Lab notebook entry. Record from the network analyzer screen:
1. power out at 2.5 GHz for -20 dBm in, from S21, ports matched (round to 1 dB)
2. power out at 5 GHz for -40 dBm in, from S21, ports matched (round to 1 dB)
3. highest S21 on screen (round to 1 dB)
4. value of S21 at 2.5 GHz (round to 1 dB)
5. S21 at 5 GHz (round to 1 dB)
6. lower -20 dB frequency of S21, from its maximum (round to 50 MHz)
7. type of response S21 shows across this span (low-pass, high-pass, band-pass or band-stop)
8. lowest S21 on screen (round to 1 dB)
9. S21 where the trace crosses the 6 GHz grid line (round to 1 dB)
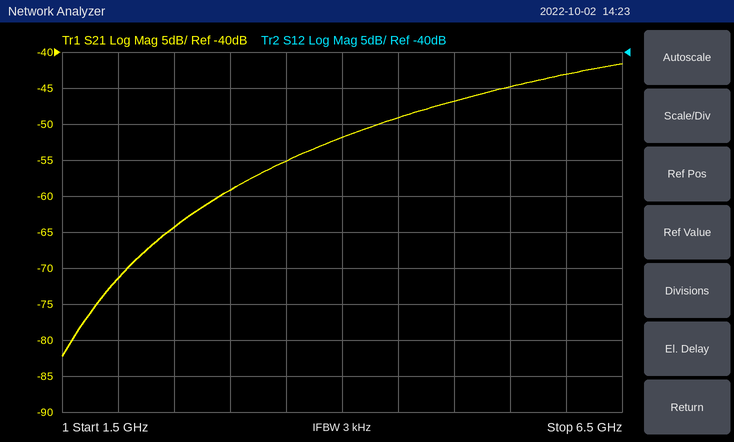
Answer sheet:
-84 dBm
-87 dBm
-42 dB
-64 dB
-47 dB
2.75 GHz
high-pass
-82 dB
-43 dB
